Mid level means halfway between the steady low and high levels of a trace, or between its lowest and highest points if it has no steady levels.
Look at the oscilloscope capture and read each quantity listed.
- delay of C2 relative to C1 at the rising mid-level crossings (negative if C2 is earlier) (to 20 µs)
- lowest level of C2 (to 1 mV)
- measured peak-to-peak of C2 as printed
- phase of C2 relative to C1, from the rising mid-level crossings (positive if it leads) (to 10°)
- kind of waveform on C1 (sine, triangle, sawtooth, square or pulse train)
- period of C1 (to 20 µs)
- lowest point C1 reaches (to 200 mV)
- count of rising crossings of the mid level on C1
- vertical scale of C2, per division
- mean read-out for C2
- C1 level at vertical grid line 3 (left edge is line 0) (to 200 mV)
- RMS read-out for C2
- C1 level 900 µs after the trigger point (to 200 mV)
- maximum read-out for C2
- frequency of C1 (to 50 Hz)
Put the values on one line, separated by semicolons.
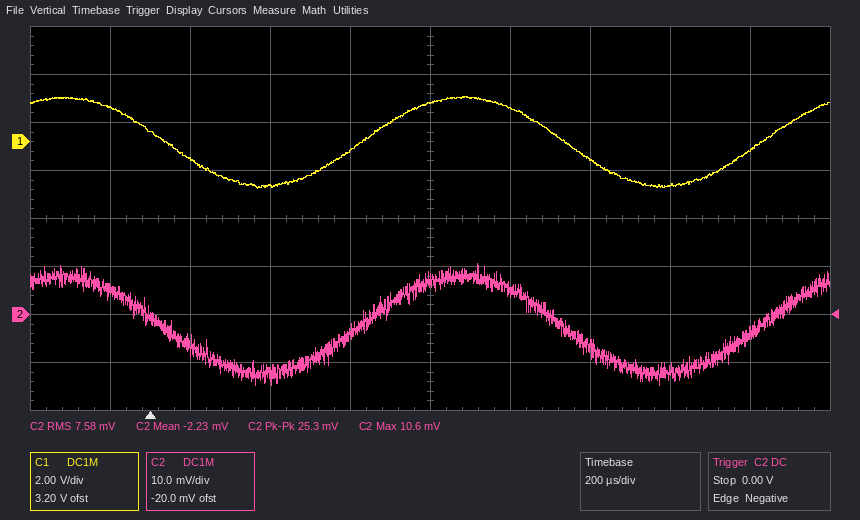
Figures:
0 µs; -15 mV; 25.3 mV; 0°; sine; 1.00 ms; -2.0 V; 2; 10 mV; -2.23 mV; -1.8 V; 7.58 mV; 1.4 V; 10.6 mV; 1.00 kHz
